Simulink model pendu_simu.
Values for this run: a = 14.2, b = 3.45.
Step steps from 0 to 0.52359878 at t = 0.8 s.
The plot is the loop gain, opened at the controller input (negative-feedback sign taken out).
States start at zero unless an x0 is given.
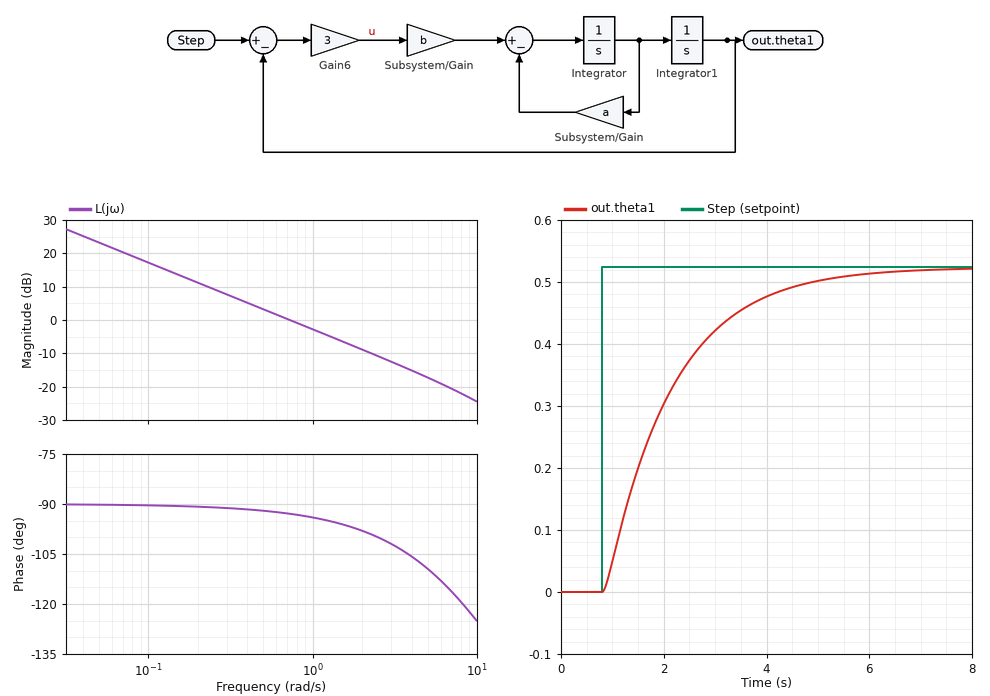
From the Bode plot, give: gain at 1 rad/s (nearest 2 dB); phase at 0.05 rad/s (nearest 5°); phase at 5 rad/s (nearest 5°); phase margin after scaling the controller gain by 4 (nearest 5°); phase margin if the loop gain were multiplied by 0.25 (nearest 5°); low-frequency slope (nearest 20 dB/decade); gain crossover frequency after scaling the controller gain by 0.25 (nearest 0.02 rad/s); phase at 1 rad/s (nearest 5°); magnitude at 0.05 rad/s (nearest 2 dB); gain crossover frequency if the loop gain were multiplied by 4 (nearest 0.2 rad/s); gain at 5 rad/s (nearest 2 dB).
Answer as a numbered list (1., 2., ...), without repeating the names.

1. -2 dB
2. -90°
3. -110°
4. 80°
5. 90°
6. -20 dB/decade
7. 0.18 rad/s
8. -95°
9. 24 dB
10. 2.8 rad/s
11. -18 dB
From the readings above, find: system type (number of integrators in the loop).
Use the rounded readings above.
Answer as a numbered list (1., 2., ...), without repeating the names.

1. 1
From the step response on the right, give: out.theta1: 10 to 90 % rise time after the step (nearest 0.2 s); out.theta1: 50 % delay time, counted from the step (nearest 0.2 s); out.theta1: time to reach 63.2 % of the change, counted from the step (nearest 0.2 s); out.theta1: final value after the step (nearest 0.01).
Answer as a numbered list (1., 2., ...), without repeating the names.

1. 2.8 s
2. 1.0 s
3. 1.4 s
4. 0.52
